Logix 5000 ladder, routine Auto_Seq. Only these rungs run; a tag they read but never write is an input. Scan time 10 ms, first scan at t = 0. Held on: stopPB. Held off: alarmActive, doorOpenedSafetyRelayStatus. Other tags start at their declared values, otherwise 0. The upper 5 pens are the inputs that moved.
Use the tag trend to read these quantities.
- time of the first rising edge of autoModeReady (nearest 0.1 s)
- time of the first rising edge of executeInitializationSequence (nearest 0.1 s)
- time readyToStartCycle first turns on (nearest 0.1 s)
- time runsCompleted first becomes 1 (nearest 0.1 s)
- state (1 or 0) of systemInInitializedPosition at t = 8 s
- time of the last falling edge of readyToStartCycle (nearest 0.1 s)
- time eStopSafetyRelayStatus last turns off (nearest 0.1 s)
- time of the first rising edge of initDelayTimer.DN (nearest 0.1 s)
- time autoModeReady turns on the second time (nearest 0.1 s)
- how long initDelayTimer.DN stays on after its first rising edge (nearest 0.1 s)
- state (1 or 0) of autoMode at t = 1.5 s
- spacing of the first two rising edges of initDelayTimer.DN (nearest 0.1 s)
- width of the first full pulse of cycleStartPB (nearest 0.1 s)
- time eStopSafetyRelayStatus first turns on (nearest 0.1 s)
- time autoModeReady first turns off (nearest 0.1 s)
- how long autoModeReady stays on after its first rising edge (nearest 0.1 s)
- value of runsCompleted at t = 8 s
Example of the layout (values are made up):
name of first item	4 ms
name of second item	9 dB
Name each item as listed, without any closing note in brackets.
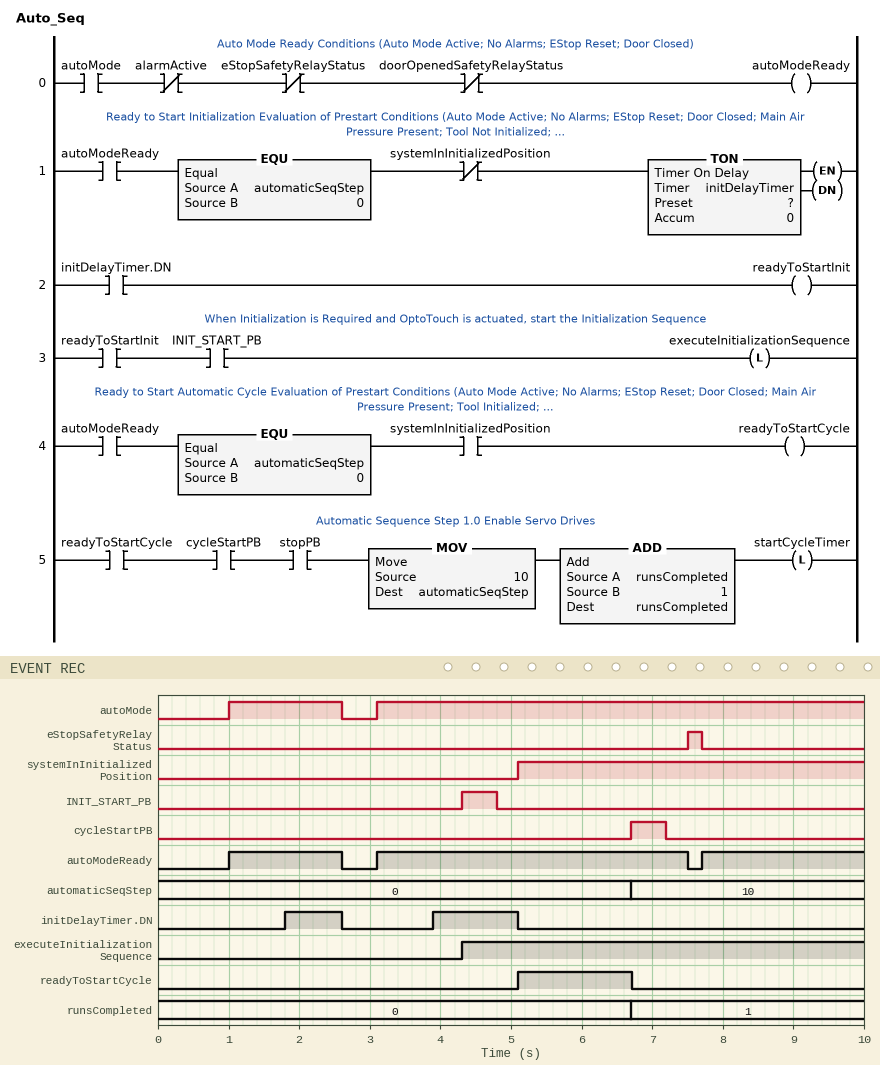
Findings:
time of the first rising edge of autoModeReady	1.0 s
time of the first rising edge of executeInitializationSequence	4.3 s
time readyToStartCycle first turns on	5.1 s
time runsCompleted first becomes 1	6.7 s
state (1 or 0) of systemInInitializedPosition at t = 8 s	1
time of the last falling edge of readyToStartCycle	6.7 s
time eStopSafetyRelayStatus last turns off	7.7 s
time of the first rising edge of initDelayTimer.DN	1.8 s
time autoModeReady turns on the second time	3.1 s
how long initDelayTimer.DN stays on after its first rising edge	0.8 s
state (1 or 0) of autoMode at t = 1.5 s	1
spacing of the first two rising edges of initDelayTimer.DN	2.1 s
width of the first full pulse of cycleStartPB	0.5 s
time eStopSafetyRelayStatus first turns on	7.5 s
time autoModeReady first turns off	2.6 s
how long autoModeReady stays on after its first rising edge	1.6 s
value of runsCompleted at t = 8 s	1
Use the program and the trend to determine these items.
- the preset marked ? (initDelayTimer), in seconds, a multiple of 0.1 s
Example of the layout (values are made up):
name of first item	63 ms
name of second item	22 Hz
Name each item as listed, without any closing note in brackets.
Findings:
the preset marked ? (initDelayTimer), in seconds, a multiple of 0.1 s	0.8 s
